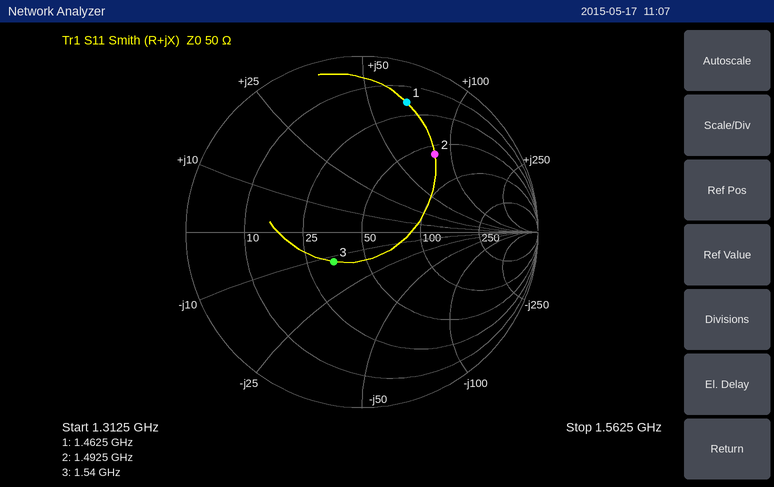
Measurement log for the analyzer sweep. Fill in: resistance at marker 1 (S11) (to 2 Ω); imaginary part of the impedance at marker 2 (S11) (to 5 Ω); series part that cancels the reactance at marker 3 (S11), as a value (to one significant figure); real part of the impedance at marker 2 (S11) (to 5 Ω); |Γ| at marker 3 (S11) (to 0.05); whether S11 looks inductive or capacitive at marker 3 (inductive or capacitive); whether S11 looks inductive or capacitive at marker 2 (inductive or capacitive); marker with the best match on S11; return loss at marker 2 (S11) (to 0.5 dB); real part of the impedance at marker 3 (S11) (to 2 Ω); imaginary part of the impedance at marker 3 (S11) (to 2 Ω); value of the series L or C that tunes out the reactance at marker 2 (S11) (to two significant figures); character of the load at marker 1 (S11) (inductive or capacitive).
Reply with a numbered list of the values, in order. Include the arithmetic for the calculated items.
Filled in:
1. 18 Ω
2. +80 Ω
3. L = 12 Ω/(2π × 1.54 GHz) ≈ 1 nH
4. 60 Ω
5. 0.25
6. capacitive
7. inductive
8. marker 3
9. 4.5 dB
10. 34 Ω
11. -12 Ω
12. C = 1/(2π × 1.4925 GHz × 80 Ω) ≈ 1.3 pF
13. inductive
